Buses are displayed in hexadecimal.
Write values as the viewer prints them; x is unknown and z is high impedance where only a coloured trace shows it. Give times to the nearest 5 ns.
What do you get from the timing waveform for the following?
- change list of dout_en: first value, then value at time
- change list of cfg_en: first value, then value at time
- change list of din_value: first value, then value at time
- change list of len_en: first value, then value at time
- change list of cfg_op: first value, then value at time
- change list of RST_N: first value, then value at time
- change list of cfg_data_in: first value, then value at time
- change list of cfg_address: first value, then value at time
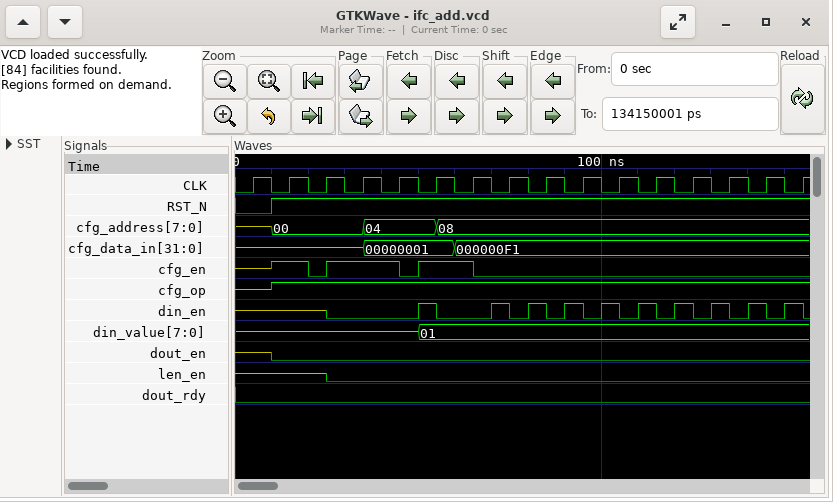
z, 0 at 10 ns
z, 1 at 10 ns, 0 at 20 ns, 1 at 25 ns, 0 at 45 ns, 1 at 50 ns, 0 at 65 ns
z, 01 at 50 ns
z, 0 at 25 ns
z, 1 at 10 ns
0, 1 at 10 ns
z, 00000001 at 35 ns, 000000F1 at 60 ns
z, 00 at 10 ns, 04 at 35 ns, 08 at 55 ns
